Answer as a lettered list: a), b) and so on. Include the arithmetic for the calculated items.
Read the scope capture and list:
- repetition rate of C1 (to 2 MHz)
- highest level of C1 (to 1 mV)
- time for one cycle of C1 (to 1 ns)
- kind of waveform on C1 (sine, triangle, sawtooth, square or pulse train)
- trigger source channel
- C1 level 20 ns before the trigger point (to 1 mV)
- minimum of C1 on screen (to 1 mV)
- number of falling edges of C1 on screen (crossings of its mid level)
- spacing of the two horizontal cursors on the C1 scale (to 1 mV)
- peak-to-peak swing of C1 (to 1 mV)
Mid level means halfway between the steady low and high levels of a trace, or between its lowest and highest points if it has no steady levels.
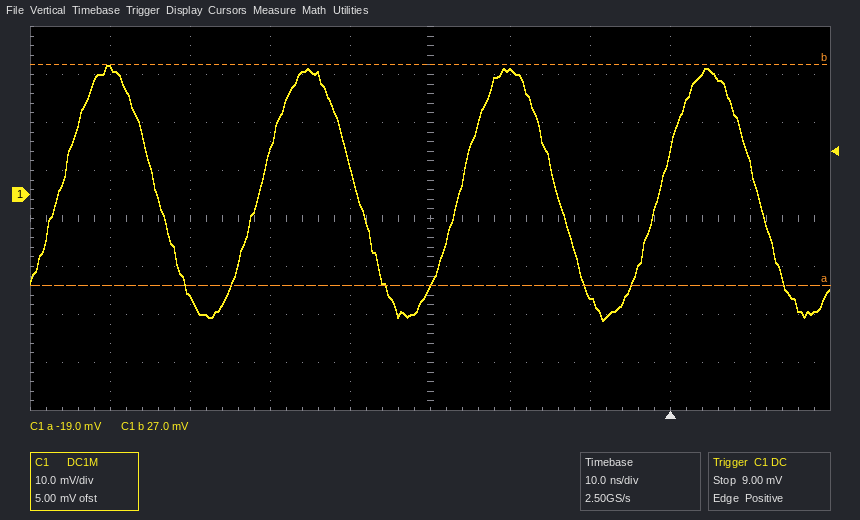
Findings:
a) 1 / 25 ns ≈ 40 MHz
b) 27 mV
c) 25 ns
d) sine
e) C1
f) 26 mV
g) -26 mV
h) 4
i) 46 mV
j) 27 mV − (-26 mV) = 53 mV
